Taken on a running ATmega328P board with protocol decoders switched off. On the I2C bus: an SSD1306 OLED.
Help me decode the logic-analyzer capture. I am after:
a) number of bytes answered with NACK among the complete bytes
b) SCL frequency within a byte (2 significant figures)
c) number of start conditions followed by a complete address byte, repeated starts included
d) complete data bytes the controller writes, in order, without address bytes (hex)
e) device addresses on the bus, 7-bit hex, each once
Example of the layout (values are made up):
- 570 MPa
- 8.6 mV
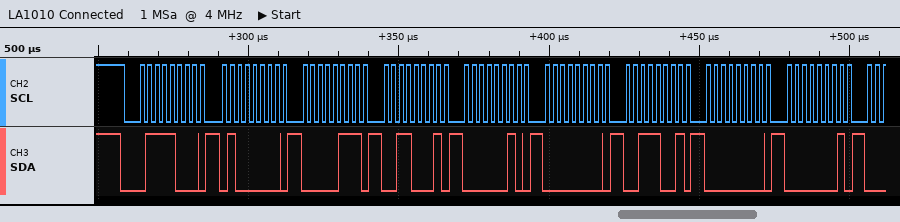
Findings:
- 0
- 400 kHz
- 1
- 40 07 31 02 00 39 00 01
- 0x3C
